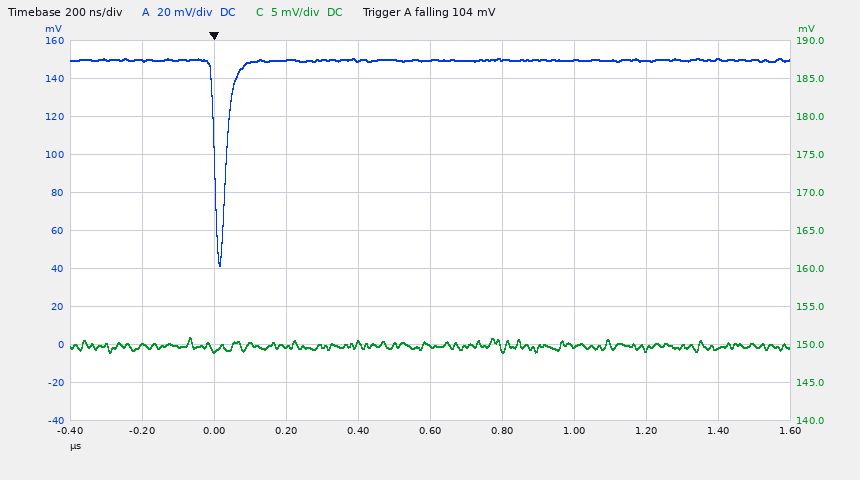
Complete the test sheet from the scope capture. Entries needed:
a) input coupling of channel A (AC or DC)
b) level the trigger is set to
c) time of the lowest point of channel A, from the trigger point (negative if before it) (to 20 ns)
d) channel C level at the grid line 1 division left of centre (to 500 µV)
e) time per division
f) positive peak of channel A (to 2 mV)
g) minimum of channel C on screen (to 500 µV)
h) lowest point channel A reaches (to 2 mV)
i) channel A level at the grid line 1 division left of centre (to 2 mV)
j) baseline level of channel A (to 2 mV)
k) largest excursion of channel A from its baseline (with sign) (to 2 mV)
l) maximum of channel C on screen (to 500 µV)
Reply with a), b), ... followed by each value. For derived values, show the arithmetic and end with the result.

a) DC
b) 104 mV
c) +20 ns
d) 150.0 mV
e) 200 ns
f) 150 mV
g) 149.0 mV
h) 42 mV
i) 150 mV
j) 150 mV
k) 42 mV − (150 mV) = -108 mV
l) 151.0 mV
